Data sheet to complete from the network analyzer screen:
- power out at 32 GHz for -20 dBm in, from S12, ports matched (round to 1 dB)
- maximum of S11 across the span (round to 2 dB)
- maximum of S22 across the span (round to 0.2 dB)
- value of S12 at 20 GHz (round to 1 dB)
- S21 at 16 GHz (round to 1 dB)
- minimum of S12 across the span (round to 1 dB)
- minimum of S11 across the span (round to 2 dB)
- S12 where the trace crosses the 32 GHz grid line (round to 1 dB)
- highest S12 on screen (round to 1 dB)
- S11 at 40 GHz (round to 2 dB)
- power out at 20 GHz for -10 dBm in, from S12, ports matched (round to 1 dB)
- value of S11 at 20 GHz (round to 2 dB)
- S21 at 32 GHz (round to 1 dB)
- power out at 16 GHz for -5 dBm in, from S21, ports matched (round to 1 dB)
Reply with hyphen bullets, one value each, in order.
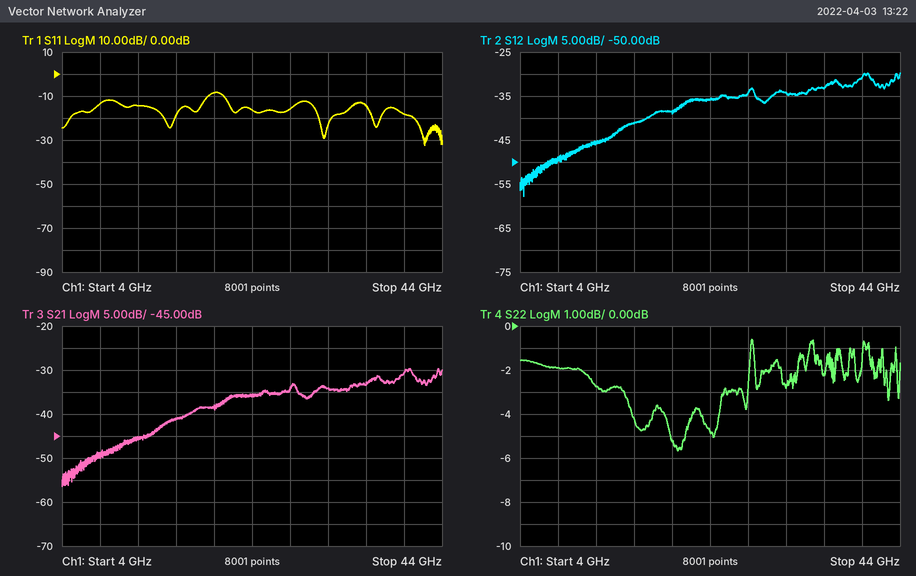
- -54 dBm
- -8 dB
- -0.6 dB
- -39 dB
- -41 dB
- -58 dB
- -32 dB
- -34 dB
- -30 dB
- -18 dB
- -49 dBm
- -8 dB
- -34 dB
- -46 dBm
